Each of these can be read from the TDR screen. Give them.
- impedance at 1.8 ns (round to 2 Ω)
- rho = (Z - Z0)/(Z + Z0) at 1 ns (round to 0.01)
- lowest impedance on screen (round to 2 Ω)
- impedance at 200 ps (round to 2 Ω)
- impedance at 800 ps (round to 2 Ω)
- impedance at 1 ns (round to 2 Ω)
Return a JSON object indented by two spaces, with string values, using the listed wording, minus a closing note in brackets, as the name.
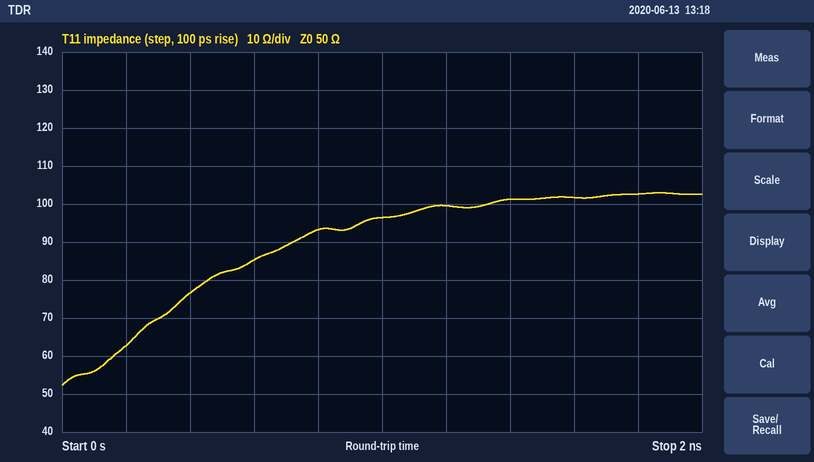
{
  "impedance at 1.8 ns": "102 Ω",
  "rho = (Z - Z0)/(Z + Z0) at 1 ns": "+0.32",
  "lowest impedance on screen": "52 Ω",
  "impedance at 200 ps": "62 Ω",
  "impedance at 800 ps": "94 Ω",
  "impedance at 1 ns": "96 Ω"
}
